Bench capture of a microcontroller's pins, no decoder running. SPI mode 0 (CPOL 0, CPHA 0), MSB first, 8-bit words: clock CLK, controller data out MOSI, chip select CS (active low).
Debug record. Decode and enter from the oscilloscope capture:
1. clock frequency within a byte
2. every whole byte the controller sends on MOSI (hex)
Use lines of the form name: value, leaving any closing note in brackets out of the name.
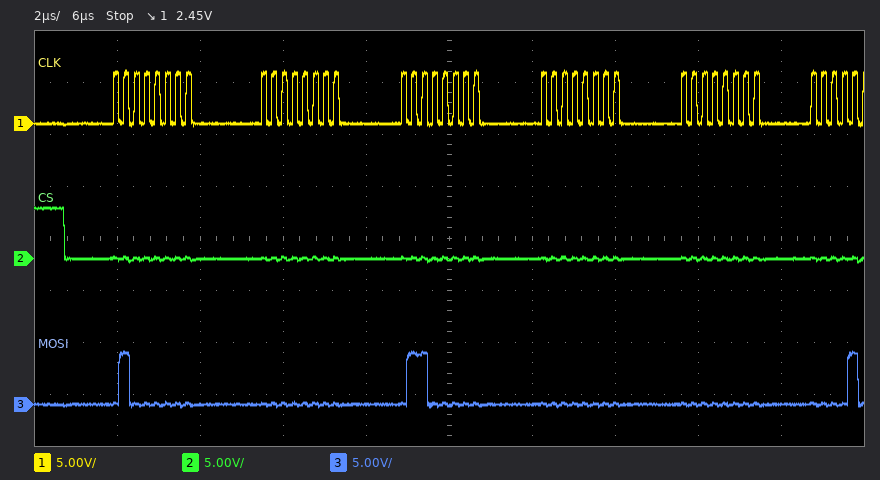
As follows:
clock frequency within a byte: 4 MHz
every whole byte the controller sends on MOSI: 40 00 60 00 00
